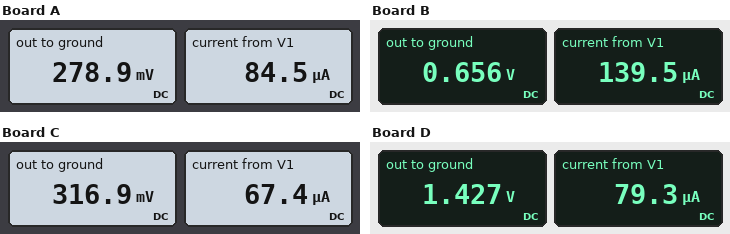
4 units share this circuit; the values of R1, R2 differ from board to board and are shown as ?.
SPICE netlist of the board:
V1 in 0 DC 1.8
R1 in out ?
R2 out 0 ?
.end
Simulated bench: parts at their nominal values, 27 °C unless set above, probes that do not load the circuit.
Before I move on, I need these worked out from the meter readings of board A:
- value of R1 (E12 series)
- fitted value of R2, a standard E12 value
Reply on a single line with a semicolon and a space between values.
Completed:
18 kΩ; 3.3 kΩ
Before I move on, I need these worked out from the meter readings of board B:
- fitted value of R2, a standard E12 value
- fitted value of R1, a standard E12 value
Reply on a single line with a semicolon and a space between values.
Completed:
4.7 kΩ; 8.2 kΩ
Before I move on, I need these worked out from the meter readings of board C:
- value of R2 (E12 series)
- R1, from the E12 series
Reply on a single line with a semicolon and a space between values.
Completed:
4.7 kΩ; 22 kΩ
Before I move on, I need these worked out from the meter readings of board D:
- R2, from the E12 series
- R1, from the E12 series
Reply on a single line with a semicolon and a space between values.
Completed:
18 kΩ; 4.7 kΩ
